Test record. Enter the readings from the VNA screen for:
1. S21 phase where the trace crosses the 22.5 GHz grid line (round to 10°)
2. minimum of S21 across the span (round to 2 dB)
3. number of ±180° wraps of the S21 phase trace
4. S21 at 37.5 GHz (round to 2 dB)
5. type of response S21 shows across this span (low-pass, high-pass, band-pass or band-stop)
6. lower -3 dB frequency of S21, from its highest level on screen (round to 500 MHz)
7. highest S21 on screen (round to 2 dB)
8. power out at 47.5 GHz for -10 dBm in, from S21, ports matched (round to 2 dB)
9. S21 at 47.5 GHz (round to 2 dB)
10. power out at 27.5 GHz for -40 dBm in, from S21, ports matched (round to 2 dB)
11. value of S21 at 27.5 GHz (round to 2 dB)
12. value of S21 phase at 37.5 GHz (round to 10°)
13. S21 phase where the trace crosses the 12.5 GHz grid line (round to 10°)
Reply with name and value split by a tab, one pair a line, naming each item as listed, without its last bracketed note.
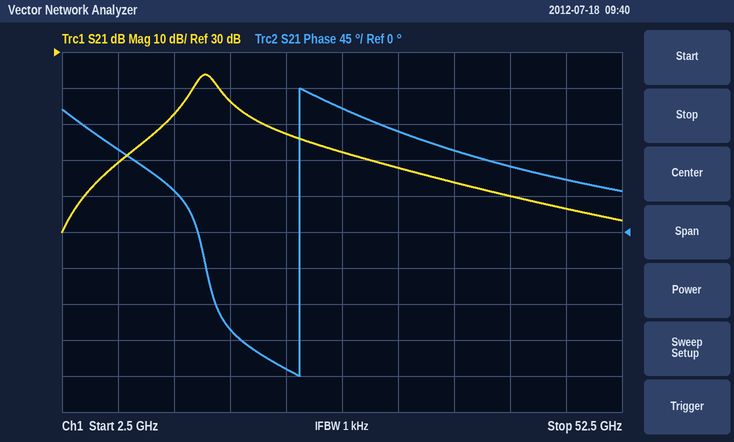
S21 phase where the trace crosses the 22.5 GHz grid line	-170°
minimum of S21 across the span	-20 dB
number of ±180° wraps of the S21 phase trace	1
S21 at 37.5 GHz	-6 dB
type of response S21 shows across this span	band-pass
lower -3 dB frequency of S21, from its highest level on screen	14.5 GHz
highest S21 on screen	24 dB
power out at 47.5 GHz for -10 dBm in, from S21, ports matched	-24 dBm
S21 at 47.5 GHz	-14 dB
power out at 27.5 GHz for -40 dBm in, from S21, ports matched	-38 dBm
value of S21 at 27.5 GHz	2 dB
value of S21 phase at 37.5 GHz	100°
S21 phase where the trace crosses the 12.5 GHz grid line	50°
